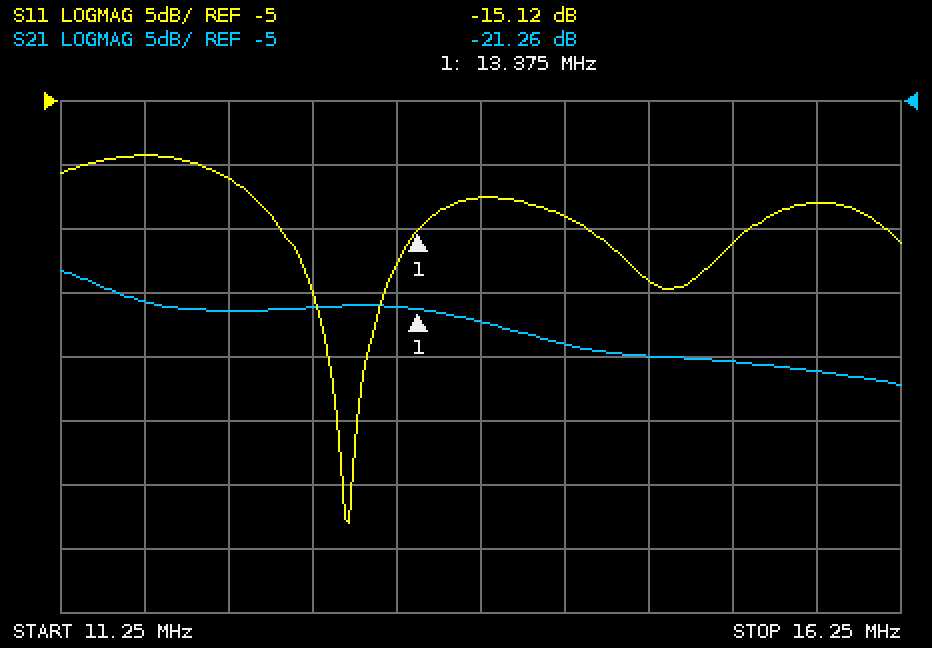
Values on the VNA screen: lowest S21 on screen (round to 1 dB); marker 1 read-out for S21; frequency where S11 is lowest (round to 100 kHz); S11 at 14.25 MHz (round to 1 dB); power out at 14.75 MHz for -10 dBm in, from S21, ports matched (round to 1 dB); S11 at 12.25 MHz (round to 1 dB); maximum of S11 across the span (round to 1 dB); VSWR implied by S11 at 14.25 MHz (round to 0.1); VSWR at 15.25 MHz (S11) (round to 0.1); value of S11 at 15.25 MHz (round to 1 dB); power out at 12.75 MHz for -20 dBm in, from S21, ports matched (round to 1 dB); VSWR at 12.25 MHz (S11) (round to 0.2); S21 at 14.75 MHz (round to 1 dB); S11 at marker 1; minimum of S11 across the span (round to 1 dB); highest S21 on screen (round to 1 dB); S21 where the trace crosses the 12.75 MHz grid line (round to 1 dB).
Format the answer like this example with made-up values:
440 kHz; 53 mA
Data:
-27 dB; -21.26 dB; 13.0 MHz; -14 dB; -35 dBm; -11 dB; -9 dB; 1.5; 1.4; -16 dB; -41 dBm; 1.8; -25 dB; -15.12 dB; -38 dB; -18 dB; -21 dB
